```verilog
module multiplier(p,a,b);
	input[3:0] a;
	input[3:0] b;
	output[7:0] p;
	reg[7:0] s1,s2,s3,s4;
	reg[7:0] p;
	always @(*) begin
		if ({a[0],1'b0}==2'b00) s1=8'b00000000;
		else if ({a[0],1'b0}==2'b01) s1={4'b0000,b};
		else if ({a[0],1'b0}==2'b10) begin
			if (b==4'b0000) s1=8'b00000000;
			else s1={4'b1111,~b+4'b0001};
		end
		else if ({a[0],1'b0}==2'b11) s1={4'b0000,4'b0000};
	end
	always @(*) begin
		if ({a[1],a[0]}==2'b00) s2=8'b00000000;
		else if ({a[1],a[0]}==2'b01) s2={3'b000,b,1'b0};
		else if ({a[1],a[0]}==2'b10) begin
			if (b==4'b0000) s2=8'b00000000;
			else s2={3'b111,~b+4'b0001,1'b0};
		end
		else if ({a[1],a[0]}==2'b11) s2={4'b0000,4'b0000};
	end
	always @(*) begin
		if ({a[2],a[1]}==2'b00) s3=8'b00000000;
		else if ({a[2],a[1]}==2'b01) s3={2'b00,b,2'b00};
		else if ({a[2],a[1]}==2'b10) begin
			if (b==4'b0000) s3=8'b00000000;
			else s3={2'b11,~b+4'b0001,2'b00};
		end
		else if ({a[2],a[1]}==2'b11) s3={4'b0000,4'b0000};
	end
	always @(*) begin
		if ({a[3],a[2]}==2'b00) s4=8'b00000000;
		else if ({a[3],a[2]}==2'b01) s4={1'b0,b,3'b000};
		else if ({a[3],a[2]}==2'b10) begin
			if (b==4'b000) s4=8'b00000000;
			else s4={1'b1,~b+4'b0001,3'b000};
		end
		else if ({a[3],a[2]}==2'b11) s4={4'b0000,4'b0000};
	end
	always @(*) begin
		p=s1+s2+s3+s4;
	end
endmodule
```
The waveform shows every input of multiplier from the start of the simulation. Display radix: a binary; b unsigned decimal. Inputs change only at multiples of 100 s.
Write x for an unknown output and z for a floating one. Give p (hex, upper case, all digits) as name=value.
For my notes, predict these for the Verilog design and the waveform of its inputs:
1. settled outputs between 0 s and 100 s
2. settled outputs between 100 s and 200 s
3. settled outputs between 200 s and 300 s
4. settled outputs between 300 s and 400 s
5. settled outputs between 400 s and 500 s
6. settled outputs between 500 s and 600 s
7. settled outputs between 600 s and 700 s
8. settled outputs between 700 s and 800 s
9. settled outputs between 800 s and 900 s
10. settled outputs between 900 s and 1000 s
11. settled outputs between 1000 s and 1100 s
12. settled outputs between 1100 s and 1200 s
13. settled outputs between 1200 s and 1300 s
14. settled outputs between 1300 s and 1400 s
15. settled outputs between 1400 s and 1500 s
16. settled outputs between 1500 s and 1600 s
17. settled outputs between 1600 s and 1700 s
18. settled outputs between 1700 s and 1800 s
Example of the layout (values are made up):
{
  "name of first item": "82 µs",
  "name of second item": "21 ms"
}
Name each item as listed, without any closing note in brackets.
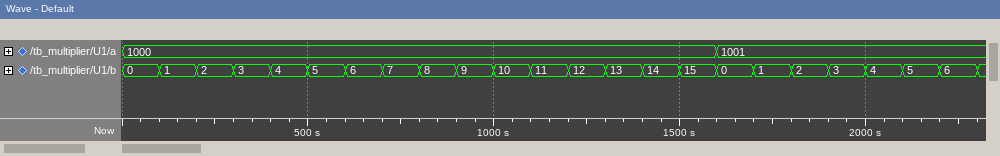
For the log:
{
  "settled outputs between 0 s and 100 s": "p=00",
  "settled outputs between 100 s and 200 s": "p=F8",
  "settled outputs between 200 s and 300 s": "p=F0",
  "settled outputs between 300 s and 400 s": "p=E8",
  "settled outputs between 400 s and 500 s": "p=E0",
  "settled outputs between 500 s and 600 s": "p=D8",
  "settled outputs between 600 s and 700 s": "p=D0",
  "settled outputs between 700 s and 800 s": "p=C8",
  "settled outputs between 800 s and 900 s": "p=C0",
  "settled outputs between 900 s and 1000 s": "p=B8",
  "settled outputs between 1000 s and 1100 s": "p=B0",
  "settled outputs between 1100 s and 1200 s": "p=A8",
  "settled outputs between 1200 s and 1300 s": "p=A0",
  "settled outputs between 1300 s and 1400 s": "p=98",
  "settled outputs between 1400 s and 1500 s": "p=90",
  "settled outputs between 1500 s and 1600 s": "p=88",
  "settled outputs between 1600 s and 1700 s": "p=00",
  "settled outputs between 1700 s and 1800 s": "p=F9"
}
